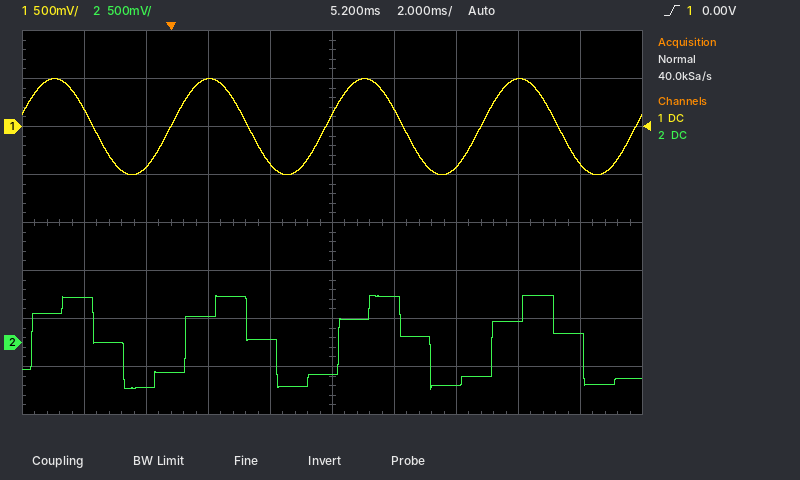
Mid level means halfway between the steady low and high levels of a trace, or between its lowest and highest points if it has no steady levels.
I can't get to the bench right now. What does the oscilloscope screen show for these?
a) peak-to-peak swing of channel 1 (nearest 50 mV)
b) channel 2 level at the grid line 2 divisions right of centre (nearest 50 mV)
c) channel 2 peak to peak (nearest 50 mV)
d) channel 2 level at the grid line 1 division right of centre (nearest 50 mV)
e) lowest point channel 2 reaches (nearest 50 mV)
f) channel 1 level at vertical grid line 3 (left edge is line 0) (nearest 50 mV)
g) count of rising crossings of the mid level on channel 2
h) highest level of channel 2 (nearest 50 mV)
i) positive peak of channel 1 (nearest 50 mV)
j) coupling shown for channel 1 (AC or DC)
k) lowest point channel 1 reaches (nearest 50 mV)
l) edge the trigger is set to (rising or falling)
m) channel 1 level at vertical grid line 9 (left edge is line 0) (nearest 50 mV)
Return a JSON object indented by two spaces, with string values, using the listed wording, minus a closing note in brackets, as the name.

{
  "peak-to-peak swing of channel 1": "1.00 V",
  "channel 2 level at the grid line 2 divisions right of centre": "-450 mV",
  "channel 2 peak to peak": "1.00 V",
  "channel 2 level at the grid line 1 division right of centre": "500 mV",
  "lowest point channel 2 reaches": "-500 mV",
  "channel 1 level at vertical grid line 3 (left edge is line 0)": "500 mV",
  "count of rising crossings of the mid level on channel 2": "4",
  "highest level of channel 2": "500 mV",
  "positive peak of channel 1": "500 mV",
  "coupling shown for channel 1": "DC",
  "lowest point channel 1 reaches": "-500 mV",
  "edge the trigger is set to": "rising",
  "channel 1 level at vertical grid line 9 (left edge is line 0)": "-400 mV"
}
